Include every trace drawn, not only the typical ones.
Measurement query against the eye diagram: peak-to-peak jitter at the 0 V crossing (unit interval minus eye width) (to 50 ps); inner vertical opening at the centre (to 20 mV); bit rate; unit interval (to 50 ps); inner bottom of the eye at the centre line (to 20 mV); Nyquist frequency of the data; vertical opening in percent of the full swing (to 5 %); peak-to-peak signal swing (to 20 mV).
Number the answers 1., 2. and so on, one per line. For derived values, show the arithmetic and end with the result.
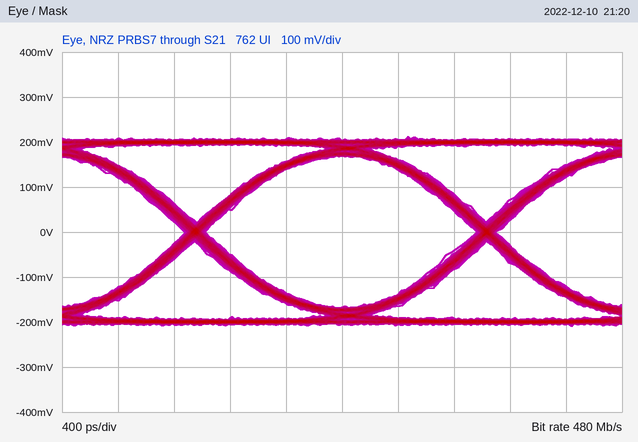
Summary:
1. 150 ps
2. 340 mV
3. 480 Mb/s
4. 2.10 ns
5. -160 mV
6. 240 MHz
7. 340 mV / 420 mV ≈ 81.0 %, so 80 % to the nearest 5 %
8. 420 mV
